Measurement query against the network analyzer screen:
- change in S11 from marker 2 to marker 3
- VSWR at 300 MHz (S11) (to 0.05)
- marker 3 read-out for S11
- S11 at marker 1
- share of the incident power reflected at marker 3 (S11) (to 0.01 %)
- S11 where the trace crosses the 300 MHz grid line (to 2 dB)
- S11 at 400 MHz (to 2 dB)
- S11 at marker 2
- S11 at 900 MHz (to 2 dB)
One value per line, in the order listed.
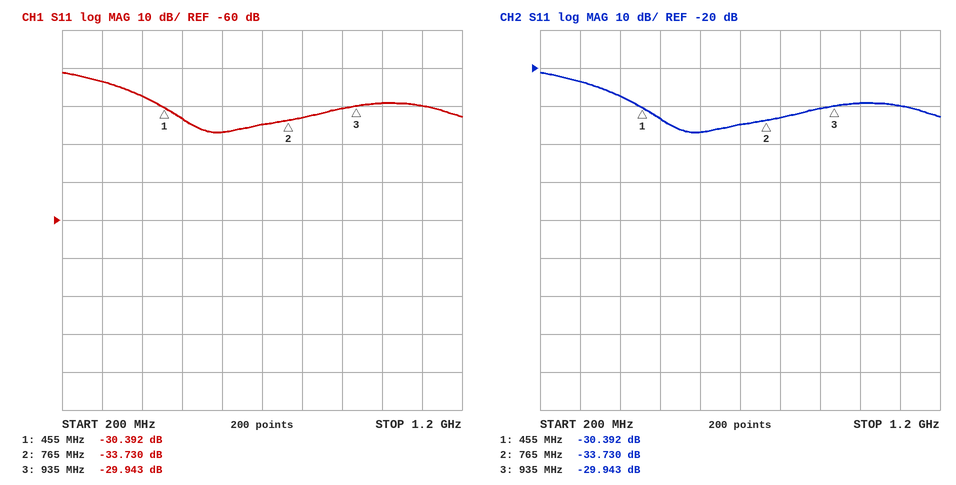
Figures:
3.787 dB
1.15
-29.943 dB
-30.392 dB
0.10 %
-24 dB
-28 dB
-33.730 dB
-30 dB
